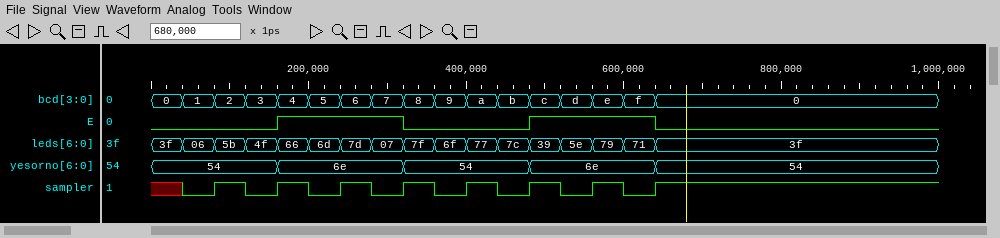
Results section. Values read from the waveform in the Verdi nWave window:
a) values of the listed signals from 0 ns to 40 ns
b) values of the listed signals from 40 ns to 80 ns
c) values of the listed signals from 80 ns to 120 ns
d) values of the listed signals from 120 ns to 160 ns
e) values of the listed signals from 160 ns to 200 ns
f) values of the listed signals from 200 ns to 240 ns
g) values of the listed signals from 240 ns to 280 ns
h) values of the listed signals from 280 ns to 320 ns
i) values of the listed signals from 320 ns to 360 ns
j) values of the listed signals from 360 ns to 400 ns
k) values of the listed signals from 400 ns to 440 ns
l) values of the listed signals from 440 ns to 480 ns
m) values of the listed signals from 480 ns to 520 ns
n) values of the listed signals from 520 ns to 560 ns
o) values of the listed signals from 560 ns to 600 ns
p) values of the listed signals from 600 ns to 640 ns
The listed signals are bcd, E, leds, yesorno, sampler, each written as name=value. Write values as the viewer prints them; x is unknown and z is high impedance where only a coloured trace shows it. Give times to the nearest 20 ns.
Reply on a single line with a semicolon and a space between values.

bcd=0, E=0, leds=3f, yesorno=54, sampler=x; bcd=1, E=0, leds=06, yesorno=54, sampler=0; bcd=2, E=0, leds=5b, yesorno=54, sampler=1; bcd=3, E=0, leds=4f, yesorno=54, sampler=0; bcd=4, E=1, leds=66, yesorno=6e, sampler=1; bcd=5, E=1, leds=6d, yesorno=6e, sampler=0; bcd=6, E=1, leds=7d, yesorno=6e, sampler=1; bcd=7, E=1, leds=07, yesorno=6e, sampler=0; bcd=8, E=0, leds=7f, yesorno=54, sampler=1; bcd=9, E=0, leds=6f, yesorno=54, sampler=0; bcd=a, E=0, leds=77, yesorno=54, sampler=1; bcd=b, E=0, leds=7c, yesorno=54, sampler=0; bcd=c, E=1, leds=39, yesorno=6e, sampler=1; bcd=d, E=1, leds=5e, yesorno=6e, sampler=0; bcd=e, E=1, leds=79, yesorno=6e, sampler=1; bcd=f, E=1, leds=71, yesorno=6e, sampler=0
